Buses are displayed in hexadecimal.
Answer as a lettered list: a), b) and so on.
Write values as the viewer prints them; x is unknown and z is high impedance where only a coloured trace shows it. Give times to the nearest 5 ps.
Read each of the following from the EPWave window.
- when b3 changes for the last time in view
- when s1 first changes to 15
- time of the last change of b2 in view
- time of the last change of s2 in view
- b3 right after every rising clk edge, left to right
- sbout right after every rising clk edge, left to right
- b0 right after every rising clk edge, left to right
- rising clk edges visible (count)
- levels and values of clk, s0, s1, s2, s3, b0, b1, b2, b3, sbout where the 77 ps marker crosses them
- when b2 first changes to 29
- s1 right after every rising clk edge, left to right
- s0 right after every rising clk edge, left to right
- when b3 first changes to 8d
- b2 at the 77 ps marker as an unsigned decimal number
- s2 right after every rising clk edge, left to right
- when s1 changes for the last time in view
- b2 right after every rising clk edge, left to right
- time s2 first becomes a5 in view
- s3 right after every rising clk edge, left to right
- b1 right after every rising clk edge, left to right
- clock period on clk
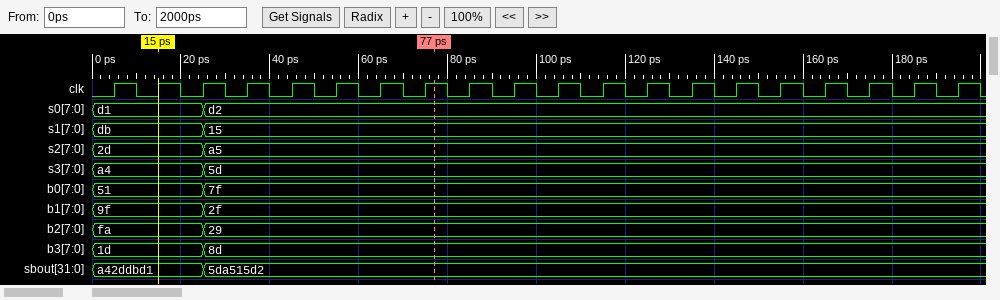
a) 25 ps
b) 25 ps
c) 25 ps
d) 25 ps
e) 1d, 1d, 8d, 8d, 8d, 8d, 8d, 8d, 8d, 8d, 8d, 8d, 8d, 8d, 8d, 8d, 8d, 8d, 8d, 8d
f) a42ddbd1, a42ddbd1, 5da515d2, 5da515d2, 5da515d2, 5da515d2, 5da515d2, 5da515d2, 5da515d2, 5da515d2, 5da515d2, 5da515d2, 5da515d2, 5da515d2, 5da515d2, 5da515d2, 5da515d2, 5da515d2, 5da515d2, 5da515d2
g) 51, 51, 7f, 7f, 7f, 7f, 7f, 7f, 7f, 7f, 7f, 7f, 7f, 7f, 7f, 7f, 7f, 7f, 7f, 7f
h) 20
i) clk=1, s0=d2, s1=15, s2=a5, s3=5d, b0=7f, b1=2f, b2=29, b3=8d, sbout=5da515d2
j) 25 ps
k) db, db, 15, 15, 15, 15, 15, 15, 15, 15, 15, 15, 15, 15, 15, 15, 15, 15, 15, 15
l) d1, d1, d2, d2, d2, d2, d2, d2, d2, d2, d2, d2, d2, d2, d2, d2, d2, d2, d2, d2
m) 25 ps
n) 41
o) 2d, 2d, a5, a5, a5, a5, a5, a5, a5, a5, a5, a5, a5, a5, a5, a5, a5, a5, a5, a5
p) 25 ps
q) fa, fa, 29, 29, 29, 29, 29, 29, 29, 29, 29, 29, 29, 29, 29, 29, 29, 29, 29, 29
r) 25 ps
s) a4, a4, 5d, 5d, 5d, 5d, 5d, 5d, 5d, 5d, 5d, 5d, 5d, 5d, 5d, 5d, 5d, 5d, 5d, 5d
t) 9f, 9f, 2f, 2f, 2f, 2f, 2f, 2f, 2f, 2f, 2f, 2f, 2f, 2f, 2f, 2f, 2f, 2f, 2f, 2f
u) 10 ps
